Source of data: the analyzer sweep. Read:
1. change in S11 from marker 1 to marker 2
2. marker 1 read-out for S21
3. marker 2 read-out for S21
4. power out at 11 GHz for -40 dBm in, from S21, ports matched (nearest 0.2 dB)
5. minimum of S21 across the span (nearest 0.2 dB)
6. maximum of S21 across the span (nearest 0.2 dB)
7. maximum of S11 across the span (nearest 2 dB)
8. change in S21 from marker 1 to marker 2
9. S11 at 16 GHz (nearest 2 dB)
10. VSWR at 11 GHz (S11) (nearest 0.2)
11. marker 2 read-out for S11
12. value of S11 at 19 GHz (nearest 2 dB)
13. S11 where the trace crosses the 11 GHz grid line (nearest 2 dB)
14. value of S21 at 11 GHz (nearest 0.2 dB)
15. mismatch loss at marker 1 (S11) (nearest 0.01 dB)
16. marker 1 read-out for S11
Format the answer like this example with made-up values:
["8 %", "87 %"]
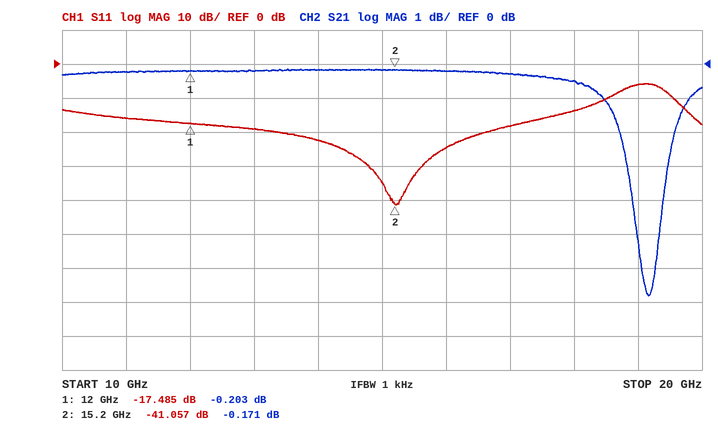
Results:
["-23.572 dB", "-0.203 dB", "-0.171 dB", "-40.2 dBm", "-6.8 dB", "-0.2 dB", "-6 dB", "0.032 dB", "-24 dB", "1.4", "-41.057 dB", "-6 dB", "-16 dB", "-0.2 dB", "0.08 dB", "-17.485 dB"]
